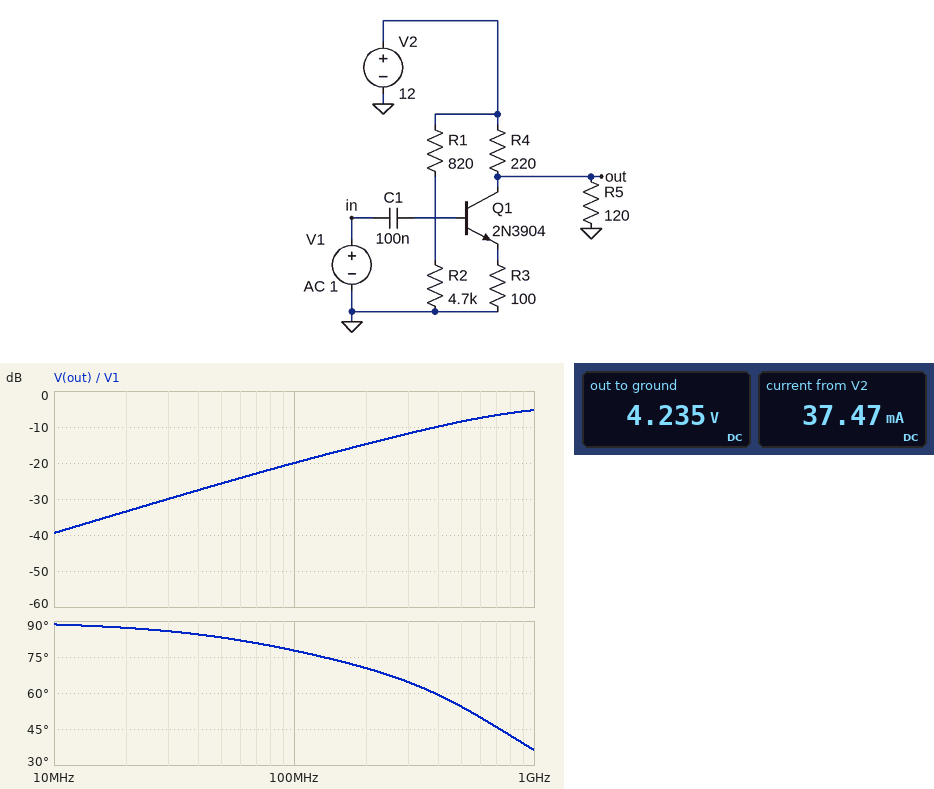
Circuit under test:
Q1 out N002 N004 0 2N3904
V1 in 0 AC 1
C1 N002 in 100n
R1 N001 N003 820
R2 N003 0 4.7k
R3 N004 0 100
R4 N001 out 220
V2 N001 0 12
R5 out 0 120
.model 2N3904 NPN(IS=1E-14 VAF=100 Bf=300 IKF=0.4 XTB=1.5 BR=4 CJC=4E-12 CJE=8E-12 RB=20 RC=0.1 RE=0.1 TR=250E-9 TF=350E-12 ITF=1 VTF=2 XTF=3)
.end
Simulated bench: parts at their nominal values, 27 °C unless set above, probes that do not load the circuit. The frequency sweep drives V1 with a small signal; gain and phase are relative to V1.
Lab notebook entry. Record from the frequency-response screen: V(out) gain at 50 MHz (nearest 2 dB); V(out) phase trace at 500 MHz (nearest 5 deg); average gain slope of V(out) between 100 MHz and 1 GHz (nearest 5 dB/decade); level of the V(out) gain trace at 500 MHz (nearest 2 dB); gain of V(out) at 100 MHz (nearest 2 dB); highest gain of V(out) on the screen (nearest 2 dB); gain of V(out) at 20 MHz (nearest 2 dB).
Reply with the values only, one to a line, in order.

-26 dB
55 deg
15 dB/decade
-8 dB
-20 dB
-6 dB
-34 dB
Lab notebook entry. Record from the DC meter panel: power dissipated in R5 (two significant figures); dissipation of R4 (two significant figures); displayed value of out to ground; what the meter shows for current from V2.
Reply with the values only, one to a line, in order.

150 mW
270 mW
4.235 V
37.47 mA
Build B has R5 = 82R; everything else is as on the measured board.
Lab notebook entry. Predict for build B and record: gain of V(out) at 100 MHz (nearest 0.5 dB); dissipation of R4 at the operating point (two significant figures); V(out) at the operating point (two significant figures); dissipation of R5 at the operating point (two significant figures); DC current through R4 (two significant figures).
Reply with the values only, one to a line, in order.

-21.5 dB
350 mW
3.3 V
130 mW
40 mA
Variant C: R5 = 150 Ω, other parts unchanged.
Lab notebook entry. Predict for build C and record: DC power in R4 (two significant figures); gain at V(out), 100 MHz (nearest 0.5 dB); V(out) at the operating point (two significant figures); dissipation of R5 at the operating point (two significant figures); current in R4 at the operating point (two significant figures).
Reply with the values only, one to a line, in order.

230 mW
-19.0 dB
4.9 V
160 mW
32 mA
